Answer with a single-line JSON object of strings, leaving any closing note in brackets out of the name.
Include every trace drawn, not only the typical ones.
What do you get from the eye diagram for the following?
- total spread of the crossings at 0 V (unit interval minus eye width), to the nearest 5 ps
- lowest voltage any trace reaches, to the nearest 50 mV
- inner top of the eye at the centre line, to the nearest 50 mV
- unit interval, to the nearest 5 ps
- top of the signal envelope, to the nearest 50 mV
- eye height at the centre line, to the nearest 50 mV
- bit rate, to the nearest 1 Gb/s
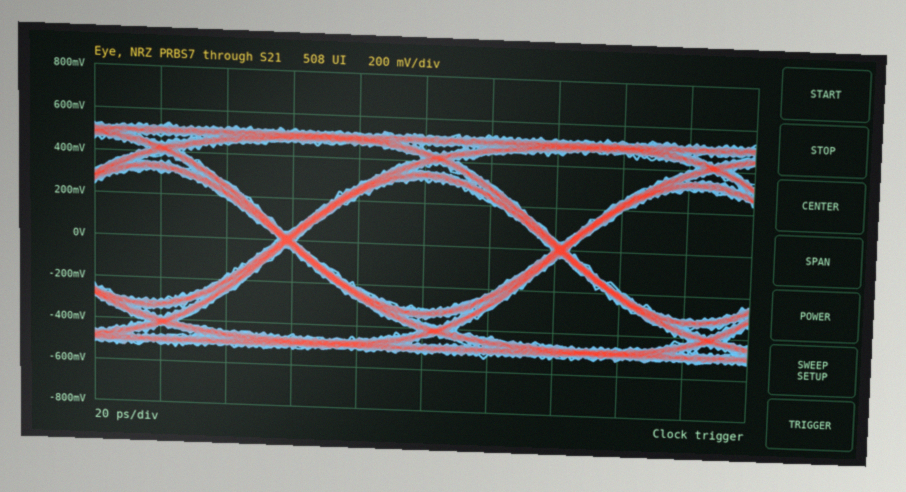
{"total spread of the crossings at 0 V (unit interval minus eye width), to the nearest 5 ps": "5 ps", "lowest voltage any trace reaches, to the nearest 50 mV": "-550 mV", "inner top of the eye at the centre line, to the nearest 50 mV": "300 mV", "unit interval, to the nearest 5 ps": "85 ps", "top of the signal envelope, to the nearest 50 mV": "550 mV", "eye height at the centre line, to the nearest 50 mV": "600 mV", "bit rate, to the nearest 1 Gb/s": "12 Gb/s"}
